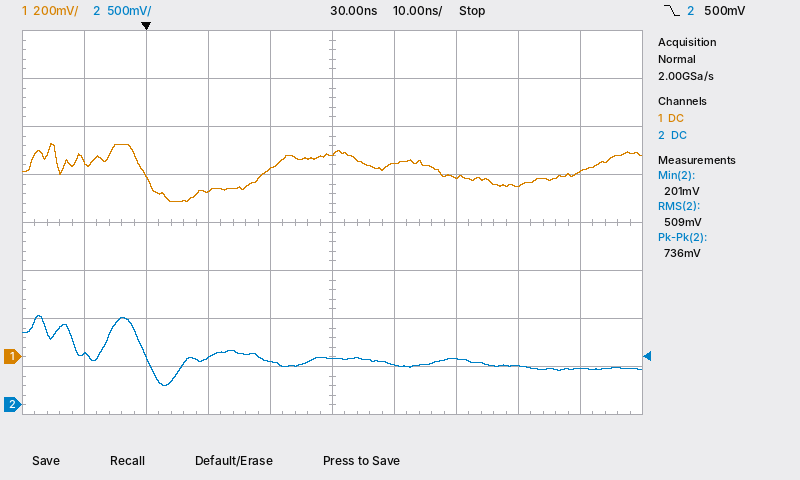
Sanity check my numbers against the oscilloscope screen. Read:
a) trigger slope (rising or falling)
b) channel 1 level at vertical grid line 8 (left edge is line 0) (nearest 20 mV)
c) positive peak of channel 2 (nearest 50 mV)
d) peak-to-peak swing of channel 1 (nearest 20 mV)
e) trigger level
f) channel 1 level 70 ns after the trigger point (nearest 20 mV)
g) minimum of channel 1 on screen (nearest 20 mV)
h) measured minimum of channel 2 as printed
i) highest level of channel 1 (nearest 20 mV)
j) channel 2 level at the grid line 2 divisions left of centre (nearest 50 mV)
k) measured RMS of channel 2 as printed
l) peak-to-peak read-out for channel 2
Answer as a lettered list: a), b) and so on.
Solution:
a) falling
b) 720 mV
c) 950 mV
d) 240 mV
e) 500 mV
f) 780 mV
g) 640 mV
h) 201 mV
i) 880 mV
j) 500 mV
k) 509 mV
l) 736 mV
